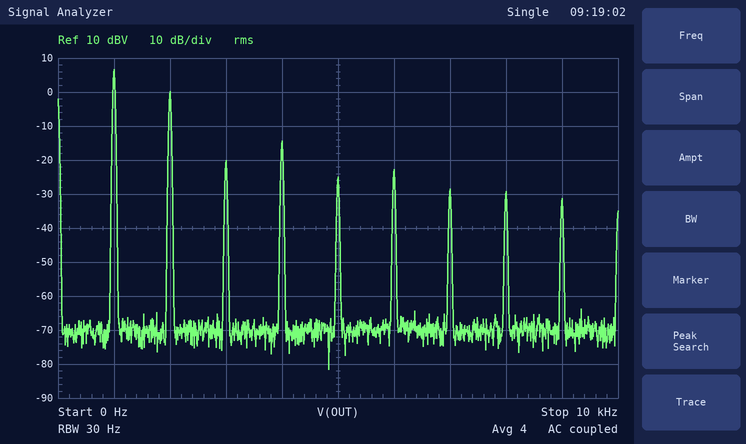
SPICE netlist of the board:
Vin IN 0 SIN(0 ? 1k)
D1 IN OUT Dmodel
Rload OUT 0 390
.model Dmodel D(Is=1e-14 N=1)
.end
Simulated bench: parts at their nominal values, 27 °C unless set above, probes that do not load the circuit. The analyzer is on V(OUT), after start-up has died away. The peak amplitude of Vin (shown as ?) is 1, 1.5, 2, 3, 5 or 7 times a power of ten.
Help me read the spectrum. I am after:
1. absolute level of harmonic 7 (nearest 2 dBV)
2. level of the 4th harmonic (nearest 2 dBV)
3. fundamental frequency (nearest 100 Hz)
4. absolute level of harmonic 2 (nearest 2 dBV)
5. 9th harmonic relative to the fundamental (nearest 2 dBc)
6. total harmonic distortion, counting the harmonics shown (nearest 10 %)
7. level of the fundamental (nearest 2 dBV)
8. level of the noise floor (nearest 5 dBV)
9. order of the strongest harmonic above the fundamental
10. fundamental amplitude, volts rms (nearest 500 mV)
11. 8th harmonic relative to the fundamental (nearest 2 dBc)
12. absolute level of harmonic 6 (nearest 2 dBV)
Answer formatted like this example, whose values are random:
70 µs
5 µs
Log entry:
-28 dBV
-14 dBV
1.0 kHz
0 dBV
-38 dBc
50 %
6 dBV
-70 dBV
2
2.0 V
-36 dBc
-22 dBV
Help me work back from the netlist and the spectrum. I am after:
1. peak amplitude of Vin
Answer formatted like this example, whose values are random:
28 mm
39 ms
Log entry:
7 V
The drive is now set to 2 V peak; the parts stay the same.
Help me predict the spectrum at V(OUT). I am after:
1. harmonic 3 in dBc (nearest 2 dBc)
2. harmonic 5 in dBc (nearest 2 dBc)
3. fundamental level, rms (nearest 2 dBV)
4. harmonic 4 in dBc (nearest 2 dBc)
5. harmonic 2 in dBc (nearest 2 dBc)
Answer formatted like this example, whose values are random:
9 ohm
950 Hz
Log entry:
-14 dBc
-22 dBc
-8 dBV
-28 dBc
-4 dBc
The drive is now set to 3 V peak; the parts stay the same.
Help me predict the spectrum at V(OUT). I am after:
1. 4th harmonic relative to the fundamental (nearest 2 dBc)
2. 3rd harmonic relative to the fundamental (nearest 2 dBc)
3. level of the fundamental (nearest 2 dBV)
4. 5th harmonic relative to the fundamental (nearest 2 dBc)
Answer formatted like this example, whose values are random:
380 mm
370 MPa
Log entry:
-22 dBc
-18 dBc
-2 dBV
-24 dBc
